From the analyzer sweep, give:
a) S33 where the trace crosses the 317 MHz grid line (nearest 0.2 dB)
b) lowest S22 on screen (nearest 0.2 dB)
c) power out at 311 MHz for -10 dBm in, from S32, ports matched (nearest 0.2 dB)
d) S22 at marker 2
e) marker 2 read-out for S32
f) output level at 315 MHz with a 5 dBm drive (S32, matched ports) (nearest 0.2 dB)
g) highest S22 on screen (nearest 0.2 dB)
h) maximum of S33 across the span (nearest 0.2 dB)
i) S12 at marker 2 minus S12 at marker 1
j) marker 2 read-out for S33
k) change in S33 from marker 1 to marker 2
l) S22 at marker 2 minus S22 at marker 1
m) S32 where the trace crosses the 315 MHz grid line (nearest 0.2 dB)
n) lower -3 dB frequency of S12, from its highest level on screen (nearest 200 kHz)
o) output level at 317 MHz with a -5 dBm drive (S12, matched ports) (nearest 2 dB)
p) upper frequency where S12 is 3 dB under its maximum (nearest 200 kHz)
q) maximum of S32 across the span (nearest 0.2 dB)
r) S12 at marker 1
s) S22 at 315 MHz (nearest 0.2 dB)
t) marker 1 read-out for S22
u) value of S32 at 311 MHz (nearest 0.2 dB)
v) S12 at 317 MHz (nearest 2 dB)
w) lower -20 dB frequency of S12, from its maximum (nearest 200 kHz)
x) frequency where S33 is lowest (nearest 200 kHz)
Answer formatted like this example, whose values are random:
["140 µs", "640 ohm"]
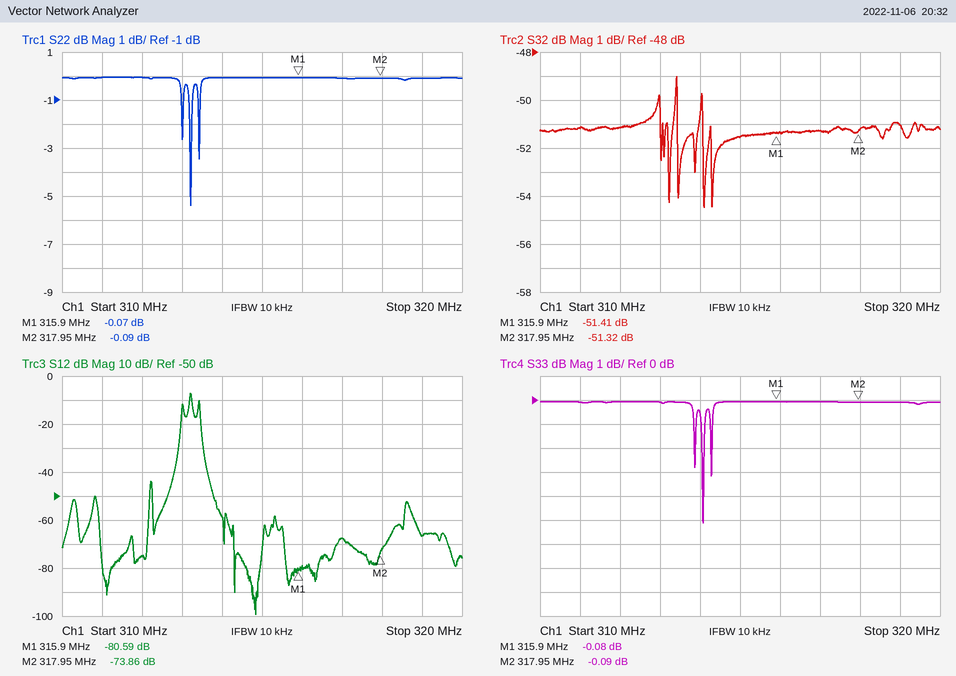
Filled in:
["0.0 dB", "-5.4 dB", "-61.2 dBm", "-0.09 dB", "-51.32 dB", "-46.6 dBm", "0.0 dB", "0.0 dB", "6.73 dB", "-0.09 dB", "-0.01 dB", "-0.02 dB", "-51.6 dB", "313.2 MHz", "-72 dBm", "313.2 MHz", "-49.0 dB", "-80.59 dB", "0.0 dB", "-0.07 dB", "-51.2 dB", "-68 dB", "313.0 MHz", "314.0 MHz"]
